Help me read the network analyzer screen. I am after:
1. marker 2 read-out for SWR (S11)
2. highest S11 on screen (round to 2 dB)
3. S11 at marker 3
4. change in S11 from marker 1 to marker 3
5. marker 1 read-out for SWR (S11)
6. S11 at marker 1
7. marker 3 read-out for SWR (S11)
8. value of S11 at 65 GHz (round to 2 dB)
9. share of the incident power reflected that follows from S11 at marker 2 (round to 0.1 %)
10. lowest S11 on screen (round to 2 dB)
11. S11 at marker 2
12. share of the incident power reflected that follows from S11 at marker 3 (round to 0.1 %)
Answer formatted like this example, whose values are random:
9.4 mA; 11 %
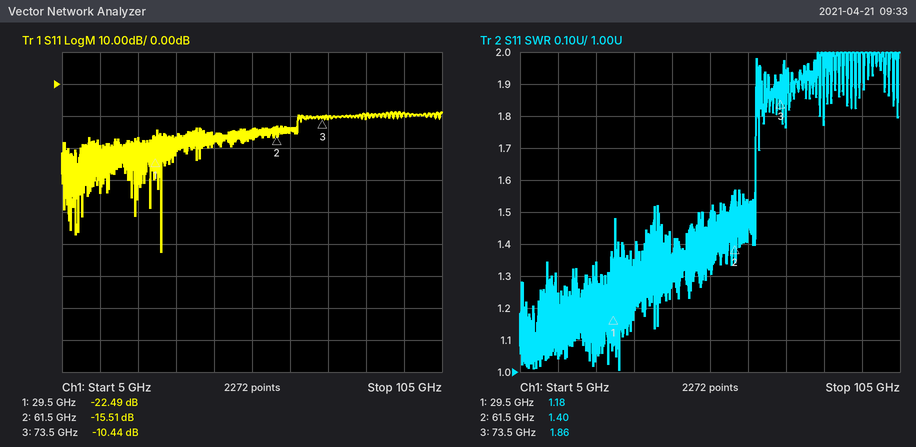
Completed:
1.40; -8 dB; -10.44 dB; 12.05 dB; 1.18; -22.49 dB; 1.86; -14 dB; 2.8 %; -52 dB; -15.51 dB; 9.0 %
